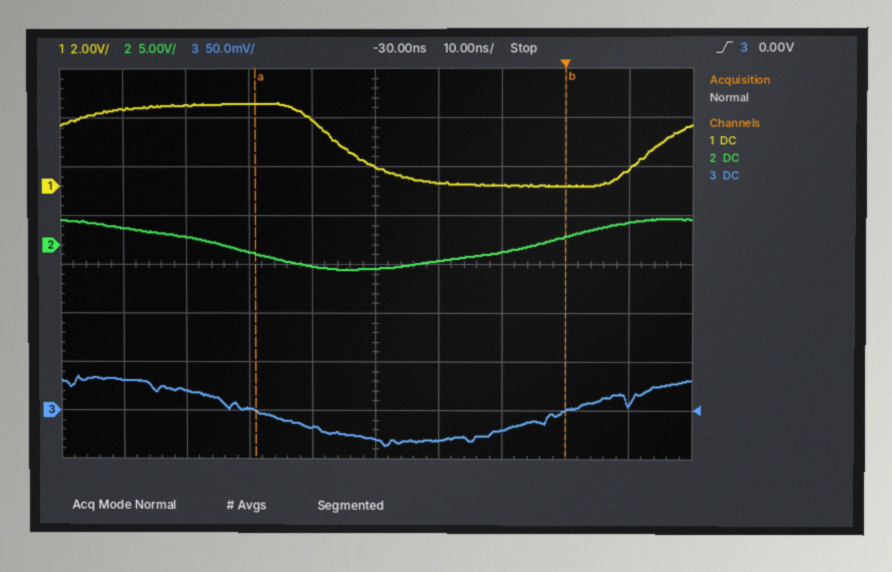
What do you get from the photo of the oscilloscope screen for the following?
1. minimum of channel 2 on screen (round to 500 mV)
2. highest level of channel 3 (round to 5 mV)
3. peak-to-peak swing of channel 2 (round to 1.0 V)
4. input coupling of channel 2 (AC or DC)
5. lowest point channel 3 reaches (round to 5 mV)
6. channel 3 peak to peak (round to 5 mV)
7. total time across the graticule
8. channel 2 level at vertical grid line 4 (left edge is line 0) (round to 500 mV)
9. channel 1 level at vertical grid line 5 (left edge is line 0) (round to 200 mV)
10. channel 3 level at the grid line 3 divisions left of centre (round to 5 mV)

-2.5 V
35 mV
5.0 V
DC
-35 mV
70 mV
100 ns
-2.0 V
800 mV
20 mV
